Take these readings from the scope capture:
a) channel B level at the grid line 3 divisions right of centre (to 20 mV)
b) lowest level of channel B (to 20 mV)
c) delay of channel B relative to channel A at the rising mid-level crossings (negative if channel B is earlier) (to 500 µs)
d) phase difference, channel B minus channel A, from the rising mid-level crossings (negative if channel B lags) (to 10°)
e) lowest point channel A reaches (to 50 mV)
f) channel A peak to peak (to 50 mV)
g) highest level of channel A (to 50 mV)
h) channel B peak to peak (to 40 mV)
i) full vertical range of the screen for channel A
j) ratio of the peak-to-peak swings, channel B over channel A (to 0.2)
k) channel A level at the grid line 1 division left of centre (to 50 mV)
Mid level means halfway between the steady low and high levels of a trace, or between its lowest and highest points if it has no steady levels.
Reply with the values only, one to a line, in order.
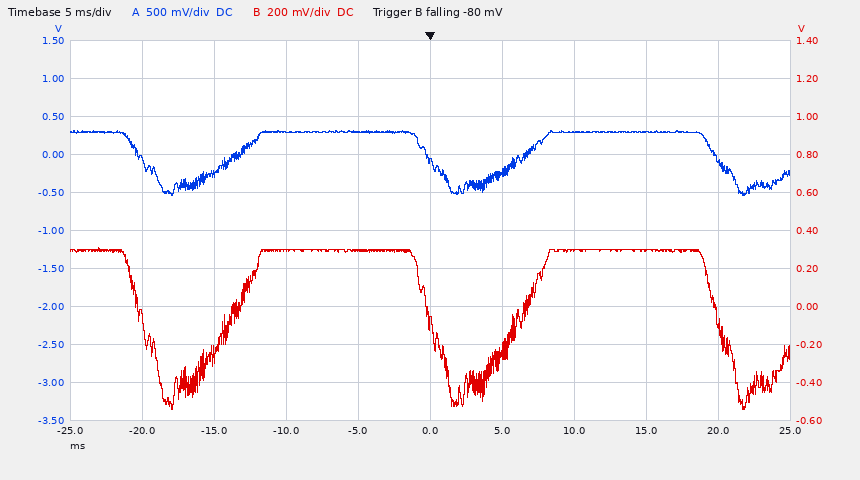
300 mV
-540 mV
0.0 ms
0°
-550 mV
850 mV
300 mV
840 mV
5 V
1.0
300 mV
